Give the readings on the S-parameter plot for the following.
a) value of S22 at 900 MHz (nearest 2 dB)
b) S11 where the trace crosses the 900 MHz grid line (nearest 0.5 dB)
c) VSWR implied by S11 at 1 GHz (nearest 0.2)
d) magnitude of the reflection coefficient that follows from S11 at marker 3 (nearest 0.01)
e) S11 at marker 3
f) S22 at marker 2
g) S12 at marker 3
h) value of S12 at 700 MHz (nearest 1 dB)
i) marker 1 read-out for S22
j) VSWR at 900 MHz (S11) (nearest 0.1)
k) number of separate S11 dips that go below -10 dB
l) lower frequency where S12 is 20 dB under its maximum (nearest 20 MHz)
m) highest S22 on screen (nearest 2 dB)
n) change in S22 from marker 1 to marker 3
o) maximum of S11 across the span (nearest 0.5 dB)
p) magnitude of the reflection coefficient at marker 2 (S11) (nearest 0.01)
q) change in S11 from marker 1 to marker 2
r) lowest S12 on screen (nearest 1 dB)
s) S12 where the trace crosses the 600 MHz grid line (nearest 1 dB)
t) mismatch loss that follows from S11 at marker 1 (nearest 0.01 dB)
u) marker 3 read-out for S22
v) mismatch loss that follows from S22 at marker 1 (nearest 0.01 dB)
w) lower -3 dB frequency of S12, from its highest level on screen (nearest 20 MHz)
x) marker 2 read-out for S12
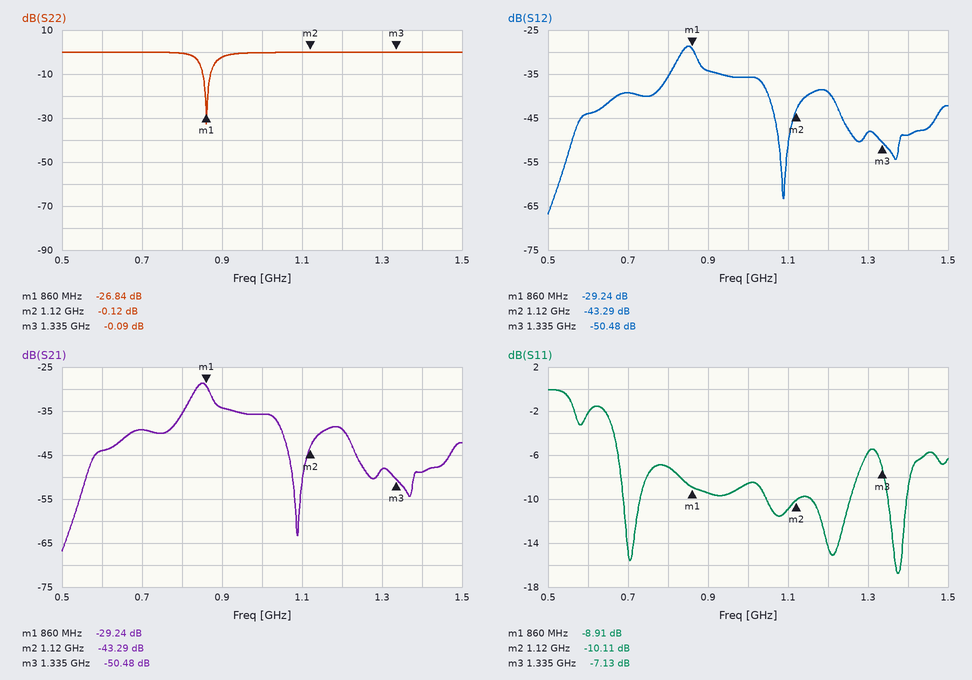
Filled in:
-2 dB
-9.5 dB
2.2
0.44
-7.13 dB
-0.12 dB
-50.48 dB
-39 dB
-26.84 dB
2.0
3
560 MHz
0 dB
26.75 dB
0.0 dB
0.31
-1.20 dB
-67 dB
-44 dB
0.60 dB
-0.09 dB
0.01 dB
820 MHz
-43.29 dB
